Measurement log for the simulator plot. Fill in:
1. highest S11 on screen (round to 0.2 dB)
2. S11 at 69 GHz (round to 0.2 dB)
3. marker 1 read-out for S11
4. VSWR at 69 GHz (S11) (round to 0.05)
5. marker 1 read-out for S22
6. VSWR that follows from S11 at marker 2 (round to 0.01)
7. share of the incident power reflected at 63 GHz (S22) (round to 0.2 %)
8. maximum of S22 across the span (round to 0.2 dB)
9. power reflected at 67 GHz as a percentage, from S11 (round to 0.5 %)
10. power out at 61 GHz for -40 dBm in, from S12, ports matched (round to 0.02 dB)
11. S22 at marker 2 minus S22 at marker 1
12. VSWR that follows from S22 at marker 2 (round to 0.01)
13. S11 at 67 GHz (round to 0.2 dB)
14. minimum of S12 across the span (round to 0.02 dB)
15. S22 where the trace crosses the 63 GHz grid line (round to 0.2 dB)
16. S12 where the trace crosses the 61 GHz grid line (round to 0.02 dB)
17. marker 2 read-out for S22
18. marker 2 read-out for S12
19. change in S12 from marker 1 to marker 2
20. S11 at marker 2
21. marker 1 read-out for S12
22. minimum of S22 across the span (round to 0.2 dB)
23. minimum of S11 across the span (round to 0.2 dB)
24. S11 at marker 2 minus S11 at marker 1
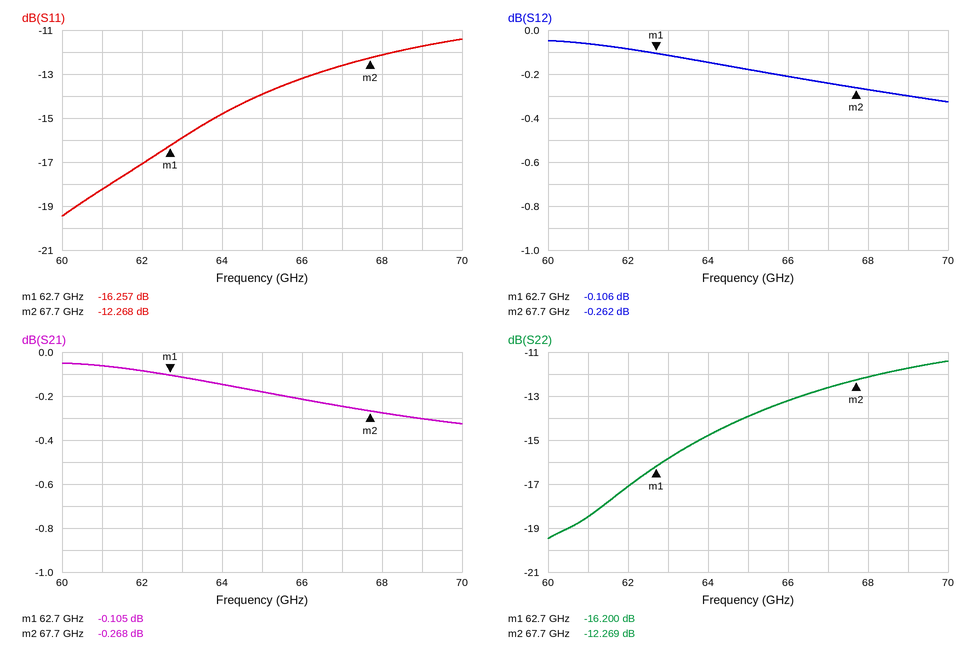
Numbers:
-11.4 dB
-11.8 dB
-16.257 dB
1.70
-16.200 dB
1.64
2.6 %
-11.4 dB
5.5 %
-40.06 dBm
3.931 dB
1.64
-12.6 dB
-0.32 dB
-15.8 dB
-0.06 dB
-12.269 dB
-0.262 dB
-0.156 dB
-12.268 dB
-0.106 dB
-19.4 dB
-19.4 dB
3.989 dB
